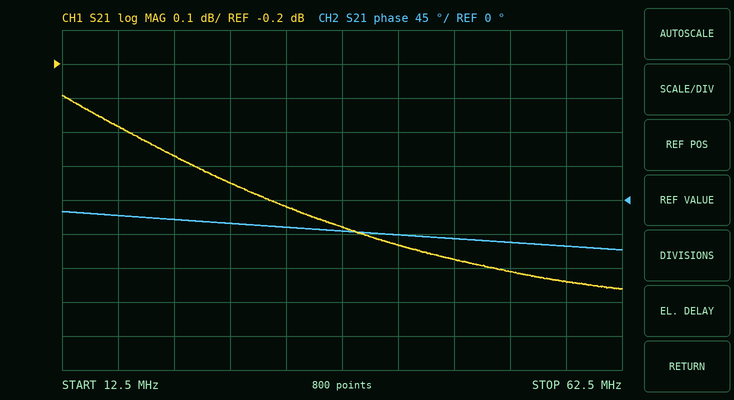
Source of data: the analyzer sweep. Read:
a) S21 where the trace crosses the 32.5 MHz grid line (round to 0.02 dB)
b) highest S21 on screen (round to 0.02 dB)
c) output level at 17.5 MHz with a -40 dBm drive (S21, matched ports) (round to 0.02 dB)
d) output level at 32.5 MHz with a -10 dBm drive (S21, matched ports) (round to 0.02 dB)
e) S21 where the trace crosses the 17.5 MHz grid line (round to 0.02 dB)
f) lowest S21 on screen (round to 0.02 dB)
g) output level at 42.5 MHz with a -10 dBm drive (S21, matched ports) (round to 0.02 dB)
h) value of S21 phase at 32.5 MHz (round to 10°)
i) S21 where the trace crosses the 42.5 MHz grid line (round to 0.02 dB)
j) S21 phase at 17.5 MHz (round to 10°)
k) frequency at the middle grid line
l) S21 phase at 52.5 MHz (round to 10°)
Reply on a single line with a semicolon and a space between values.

-0.62 dB; -0.30 dB; -40.38 dBm; -10.62 dBm; -0.38 dB; -0.86 dB; -10.74 dBm; -40°; -0.74 dB; -20°; 37.5 MHz; -60°
